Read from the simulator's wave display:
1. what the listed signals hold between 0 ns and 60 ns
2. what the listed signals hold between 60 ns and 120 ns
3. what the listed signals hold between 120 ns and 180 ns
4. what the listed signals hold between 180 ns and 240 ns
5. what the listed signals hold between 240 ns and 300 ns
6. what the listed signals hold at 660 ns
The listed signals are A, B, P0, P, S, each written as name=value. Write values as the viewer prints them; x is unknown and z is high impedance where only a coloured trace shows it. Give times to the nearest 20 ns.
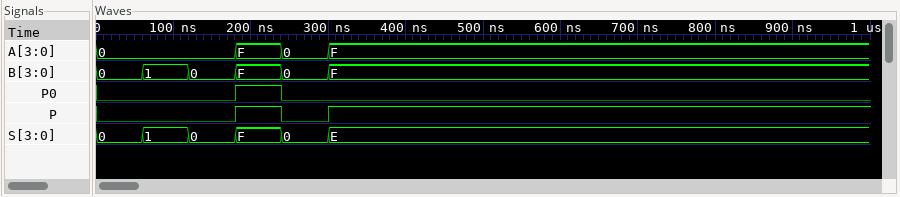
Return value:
A=0, B=0, P0=0, P=0, S=0
A=0, B=1, P0=0, P=0, S=1
A=0, B=0, P0=0, P=0, S=0
A=F, B=F, P0=1, P=1, S=F
A=0, B=0, P0=0, P=0, S=0
A=F, B=F, P0=0, P=1, S=E
